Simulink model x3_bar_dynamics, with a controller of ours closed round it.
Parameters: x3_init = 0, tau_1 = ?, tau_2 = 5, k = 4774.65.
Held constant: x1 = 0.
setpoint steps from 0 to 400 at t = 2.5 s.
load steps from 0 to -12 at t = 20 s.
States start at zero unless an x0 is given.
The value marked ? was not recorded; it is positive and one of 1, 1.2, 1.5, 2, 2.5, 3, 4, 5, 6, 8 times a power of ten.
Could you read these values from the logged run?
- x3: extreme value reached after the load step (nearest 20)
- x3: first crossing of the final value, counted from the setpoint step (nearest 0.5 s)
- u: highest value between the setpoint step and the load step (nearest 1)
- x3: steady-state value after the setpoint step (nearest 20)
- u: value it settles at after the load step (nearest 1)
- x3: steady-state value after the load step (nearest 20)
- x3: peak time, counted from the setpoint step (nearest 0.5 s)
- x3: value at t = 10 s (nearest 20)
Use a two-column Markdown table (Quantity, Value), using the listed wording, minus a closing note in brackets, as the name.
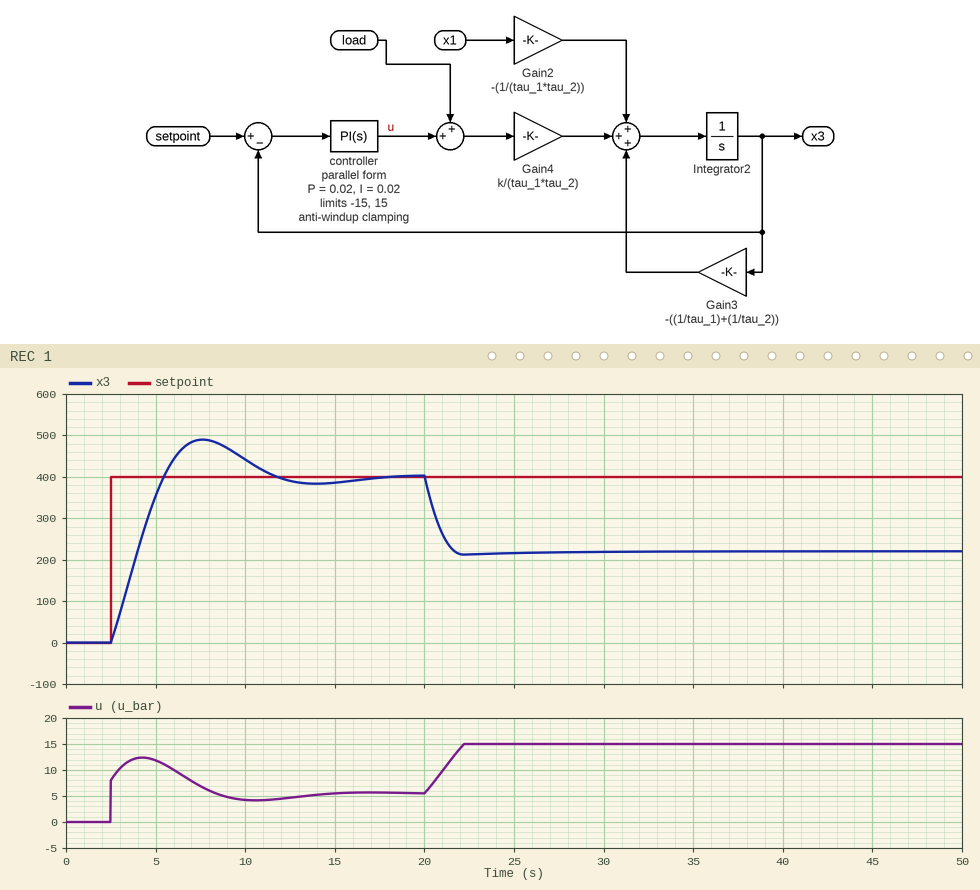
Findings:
| Quantity | Value |
|---|---|
| x3: extreme value reached after the load step | 220 |
| x3: first crossing of the final value, counted from the setpoint step | 3.0 s |
| u: highest value between the setpoint step and the load step | 12 |
| x3: steady-state value after the setpoint step | 400 |
| u: value it settles at after the load step | 15 |
| x3: steady-state value after the load step | 220 |
| x3: peak time, counted from the setpoint step | 5.0 s |
| x3: value at t = 10 s | 440 |
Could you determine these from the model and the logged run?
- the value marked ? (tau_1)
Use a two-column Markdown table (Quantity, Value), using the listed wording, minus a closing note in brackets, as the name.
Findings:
| Quantity | Value |
|---|---|
| the value marked ? | 60 |
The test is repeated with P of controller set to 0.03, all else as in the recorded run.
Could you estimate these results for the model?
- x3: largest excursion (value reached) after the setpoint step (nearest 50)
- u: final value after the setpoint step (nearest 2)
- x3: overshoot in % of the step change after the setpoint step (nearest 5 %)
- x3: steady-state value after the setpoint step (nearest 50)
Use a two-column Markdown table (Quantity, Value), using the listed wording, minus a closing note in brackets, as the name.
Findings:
| Quantity | Value |
|---|---|
| x3: largest excursion (value reached) after the setpoint step | 450 |
| u: final value after the setpoint step | 6 |
| x3: overshoot in % of the step change after the setpoint step | 15 % |
| x3: steady-state value after the setpoint step | 400 |
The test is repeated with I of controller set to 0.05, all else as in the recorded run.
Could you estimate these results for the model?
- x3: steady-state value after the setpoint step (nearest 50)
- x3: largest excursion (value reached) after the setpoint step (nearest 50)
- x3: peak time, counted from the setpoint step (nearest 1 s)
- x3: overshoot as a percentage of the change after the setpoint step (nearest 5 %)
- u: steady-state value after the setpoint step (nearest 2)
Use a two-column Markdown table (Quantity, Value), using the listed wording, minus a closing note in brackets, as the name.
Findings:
| Quantity | Value |
|---|---|
| x3: steady-state value after the setpoint step | 400 |
| x3: largest excursion (value reached) after the setpoint step | 500 |
| x3: peak time, counted from the setpoint step | 4 s |
| x3: overshoot as a percentage of the change after the setpoint step | 25 % |
| u: steady-state value after the setpoint step | 6 |
